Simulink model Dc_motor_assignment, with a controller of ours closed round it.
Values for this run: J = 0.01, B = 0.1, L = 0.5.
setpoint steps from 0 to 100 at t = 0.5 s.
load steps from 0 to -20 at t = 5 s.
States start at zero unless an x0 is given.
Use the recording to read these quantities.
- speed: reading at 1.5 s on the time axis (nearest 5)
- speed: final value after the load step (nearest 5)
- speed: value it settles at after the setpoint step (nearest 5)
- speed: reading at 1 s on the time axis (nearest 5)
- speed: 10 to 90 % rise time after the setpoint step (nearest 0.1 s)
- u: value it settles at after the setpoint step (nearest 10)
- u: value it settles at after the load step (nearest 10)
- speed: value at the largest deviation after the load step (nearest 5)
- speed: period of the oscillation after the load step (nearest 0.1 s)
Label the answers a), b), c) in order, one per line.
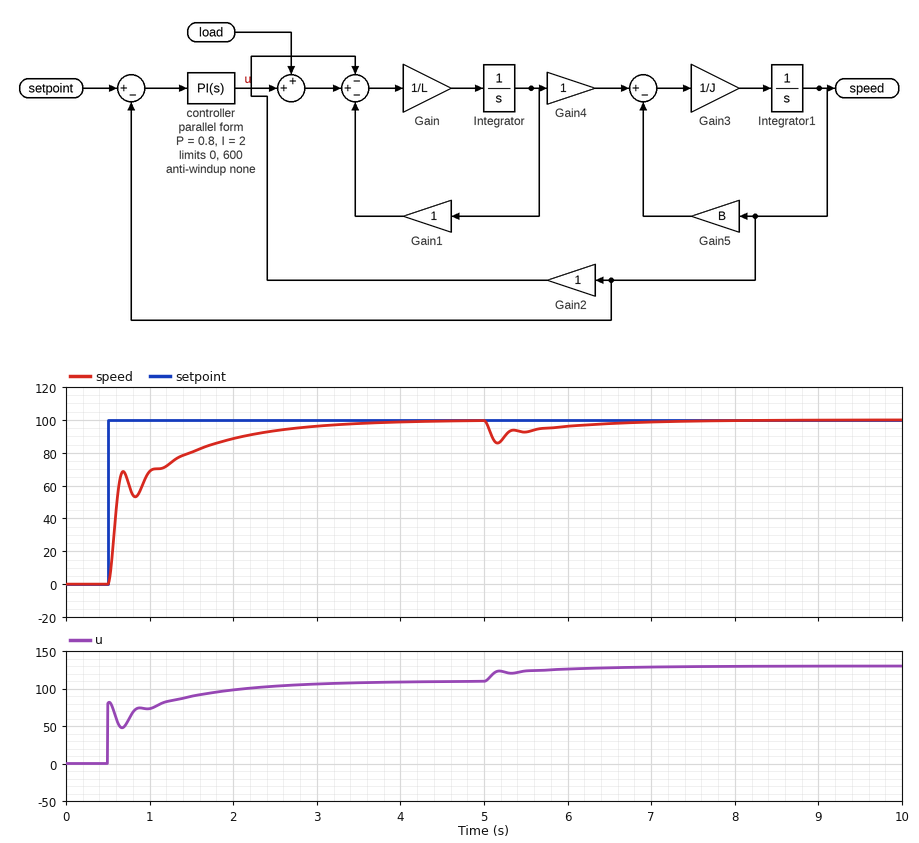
a) 80
b) 100
c) 100
d) 70
e) 1.6 s
f) 110
g) 130
h) 85
i) 0.3 s
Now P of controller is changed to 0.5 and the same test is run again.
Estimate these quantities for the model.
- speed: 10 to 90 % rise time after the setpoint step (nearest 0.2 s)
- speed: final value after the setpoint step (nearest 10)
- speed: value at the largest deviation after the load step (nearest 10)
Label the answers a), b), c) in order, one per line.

a) 1.4 s
b) 100
c) 80
